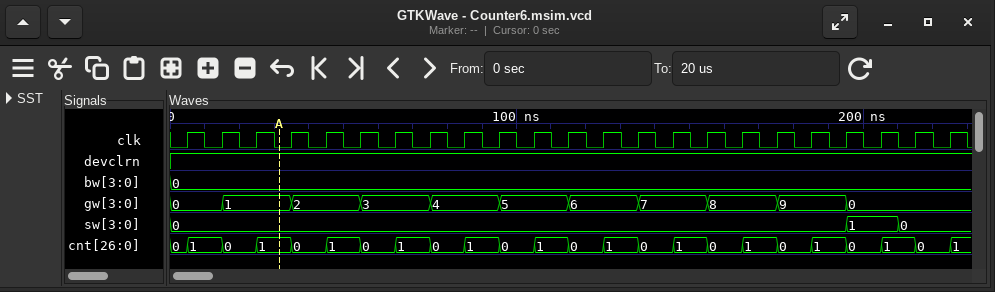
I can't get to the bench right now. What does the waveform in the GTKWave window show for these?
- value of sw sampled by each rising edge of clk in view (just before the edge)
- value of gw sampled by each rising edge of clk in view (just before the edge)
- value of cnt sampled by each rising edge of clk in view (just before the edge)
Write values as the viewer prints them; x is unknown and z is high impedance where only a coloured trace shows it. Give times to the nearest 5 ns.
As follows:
0, 0, 0, 0, 0, 0, 0, 0, 0, 0, 0, 0, 0, 0, 0, 0, 0, 0, 0, 0, 1, 0, 0
0, 0, 1, 1, 2, 2, 3, 3, 4, 4, 5, 5, 6, 6, 7, 7, 8, 8, 9, 9, 0, 0, 0
0, 1, 0, 1, 0, 1, 0, 1, 0, 1, 0, 1, 0, 1, 0, 1, 0, 1, 0, 1, 0, 1, 0
